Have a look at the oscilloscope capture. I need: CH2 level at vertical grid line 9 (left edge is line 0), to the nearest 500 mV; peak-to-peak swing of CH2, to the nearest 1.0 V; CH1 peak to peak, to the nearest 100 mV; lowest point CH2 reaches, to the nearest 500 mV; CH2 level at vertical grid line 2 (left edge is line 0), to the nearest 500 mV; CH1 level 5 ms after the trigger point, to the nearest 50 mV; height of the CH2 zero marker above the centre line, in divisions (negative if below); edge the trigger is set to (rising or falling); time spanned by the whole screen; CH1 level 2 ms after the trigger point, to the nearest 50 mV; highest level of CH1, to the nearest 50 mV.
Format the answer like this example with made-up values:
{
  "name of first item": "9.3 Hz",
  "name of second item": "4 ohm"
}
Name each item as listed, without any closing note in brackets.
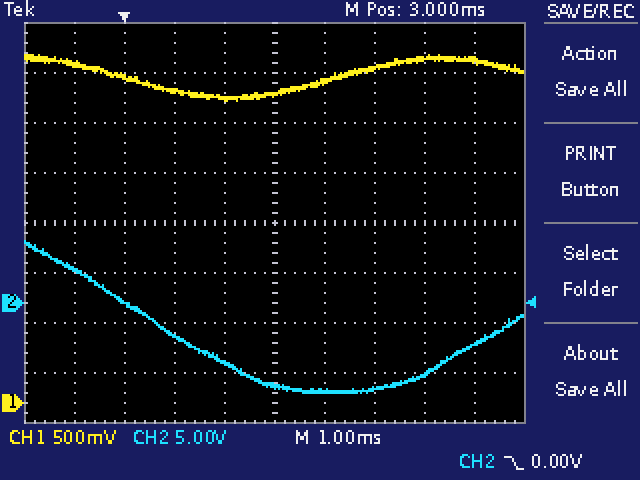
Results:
{
  "CH2 level at vertical grid line 9 (left edge is line 0), to the nearest 500 mV": "-4.0 V",
  "peak-to-peak swing of CH2, to the nearest 1.0 V": "15.0 V",
  "CH1 peak to peak, to the nearest 100 mV": "500 mV",
  "lowest point CH2 reaches, to the nearest 500 mV": "-9.0 V",
  "CH2 level at vertical grid line 2 (left edge is line 0), to the nearest 500 mV": "0.0 V",
  "CH1 level 5 ms after the trigger point, to the nearest 50 mV": "3.35 V",
  "height of the CH2 zero marker above the centre line, in divisions": "-1.6 div",
  "edge the trigger is set to": "falling",
  "time spanned by the whole screen": "10 ms",
  "CH1 level 2 ms after the trigger point, to the nearest 50 mV": "3.05 V",
  "highest level of CH1, to the nearest 50 mV": "3.50 V"
}
